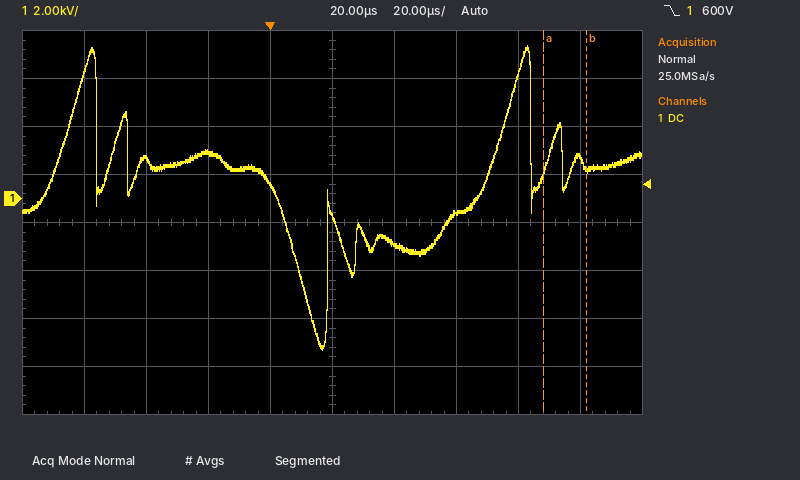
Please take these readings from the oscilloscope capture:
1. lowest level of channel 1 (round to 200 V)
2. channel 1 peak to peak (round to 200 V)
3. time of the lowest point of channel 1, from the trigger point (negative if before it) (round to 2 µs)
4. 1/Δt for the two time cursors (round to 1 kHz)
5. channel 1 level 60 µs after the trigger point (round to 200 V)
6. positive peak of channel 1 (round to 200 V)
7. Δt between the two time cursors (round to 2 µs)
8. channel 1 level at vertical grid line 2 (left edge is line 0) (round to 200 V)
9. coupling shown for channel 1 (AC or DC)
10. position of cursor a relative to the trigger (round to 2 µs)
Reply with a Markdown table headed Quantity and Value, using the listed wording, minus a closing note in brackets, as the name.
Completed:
| Quantity | Value |
|---|---|
| lowest level of channel 1 | -6.2 kV |
| channel 1 peak to peak | 12.6 kV |
| time of the lowest point of channel 1, from the trigger point (negative if before it) | +16 µs |
| 1/Δt for the two time cursors | 71 kHz |
| channel 1 level 60 µs after the trigger point | -600 V |
| positive peak of channel 1 | 6.4 kV |
| Δt between the two time cursors | 14 µs |
| channel 1 level at vertical grid line 2 (left edge is line 0) | 1.6 kV |
| coupling shown for channel 1 | DC |
| position of cursor a relative to the trigger | +88 µs |
